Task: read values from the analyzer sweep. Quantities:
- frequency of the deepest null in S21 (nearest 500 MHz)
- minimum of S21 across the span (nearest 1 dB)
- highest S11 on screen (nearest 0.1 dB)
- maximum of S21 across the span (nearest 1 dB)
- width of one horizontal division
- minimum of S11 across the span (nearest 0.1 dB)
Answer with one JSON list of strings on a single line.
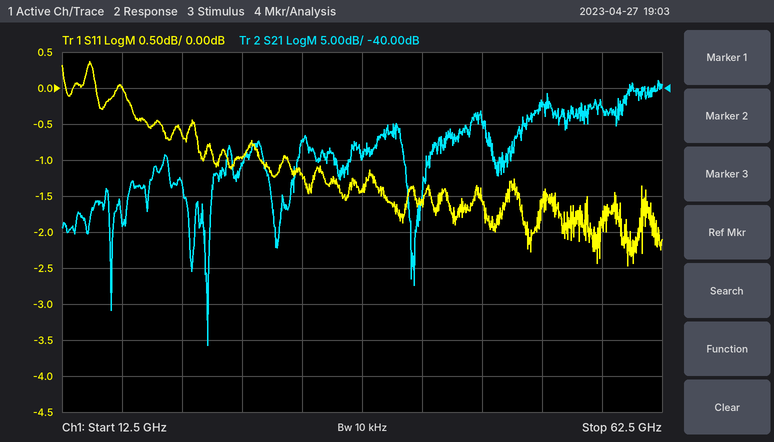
["24.5 GHz", "-76 dB", "0.4 dB", "-39 dB", "5 GHz", "-2.5 dB"]
